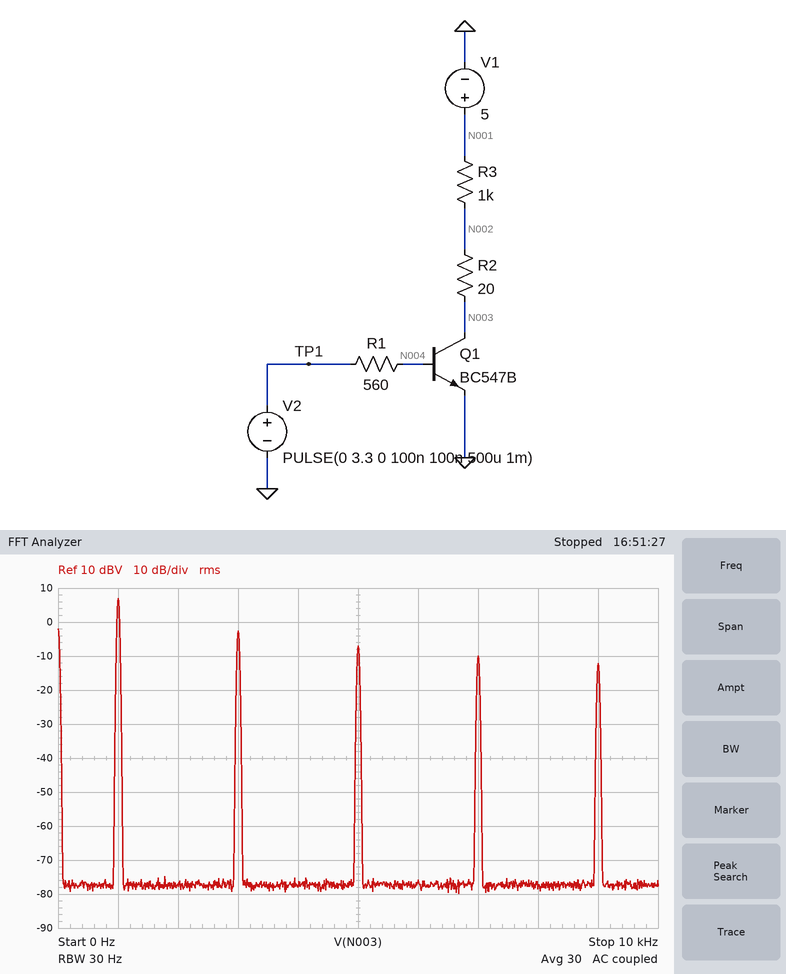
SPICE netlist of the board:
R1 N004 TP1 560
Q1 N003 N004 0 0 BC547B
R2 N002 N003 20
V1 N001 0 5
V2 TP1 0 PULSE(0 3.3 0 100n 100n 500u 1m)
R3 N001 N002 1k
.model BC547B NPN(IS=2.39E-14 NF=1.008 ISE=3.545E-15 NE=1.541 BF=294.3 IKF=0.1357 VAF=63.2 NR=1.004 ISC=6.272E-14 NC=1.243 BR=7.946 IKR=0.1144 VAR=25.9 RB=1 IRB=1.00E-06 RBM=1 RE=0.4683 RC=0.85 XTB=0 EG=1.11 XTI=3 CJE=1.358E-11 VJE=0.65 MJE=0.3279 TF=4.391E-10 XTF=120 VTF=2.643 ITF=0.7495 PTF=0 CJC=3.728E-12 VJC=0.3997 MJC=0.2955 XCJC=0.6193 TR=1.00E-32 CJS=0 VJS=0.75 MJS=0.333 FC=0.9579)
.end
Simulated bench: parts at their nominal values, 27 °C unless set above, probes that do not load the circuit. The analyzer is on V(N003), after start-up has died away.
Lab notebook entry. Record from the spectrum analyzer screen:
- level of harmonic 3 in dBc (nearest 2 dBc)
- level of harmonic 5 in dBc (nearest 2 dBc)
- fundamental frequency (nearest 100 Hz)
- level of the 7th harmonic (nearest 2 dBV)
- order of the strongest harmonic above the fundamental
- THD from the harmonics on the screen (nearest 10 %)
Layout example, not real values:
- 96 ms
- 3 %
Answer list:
- -10 dBc
- -14 dBc
- 1.0 kHz
- -10 dBV
- 3
- 40 %
